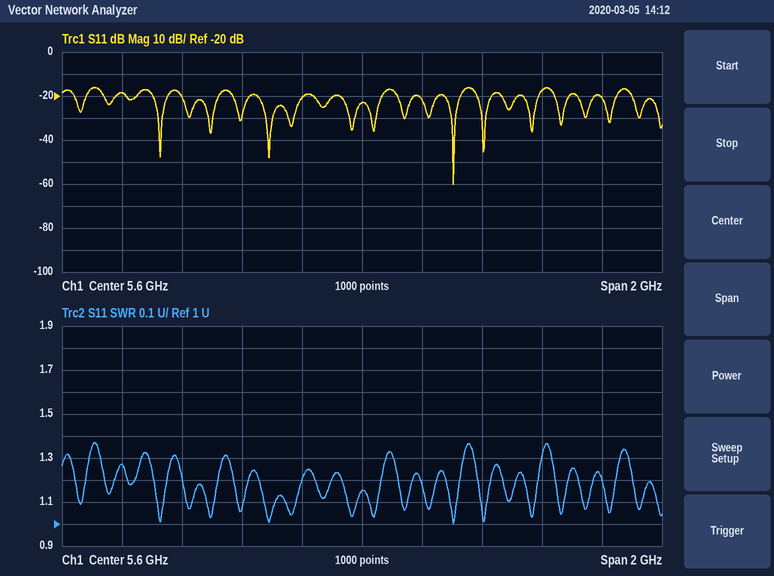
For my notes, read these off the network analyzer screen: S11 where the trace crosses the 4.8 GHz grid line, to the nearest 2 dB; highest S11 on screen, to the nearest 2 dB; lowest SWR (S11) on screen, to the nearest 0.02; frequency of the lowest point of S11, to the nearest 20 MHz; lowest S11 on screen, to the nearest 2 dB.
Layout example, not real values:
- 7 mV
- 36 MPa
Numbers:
- -18 dB
- -16 dB
- 1.00
- 5.90 GHz
- -60 dB
